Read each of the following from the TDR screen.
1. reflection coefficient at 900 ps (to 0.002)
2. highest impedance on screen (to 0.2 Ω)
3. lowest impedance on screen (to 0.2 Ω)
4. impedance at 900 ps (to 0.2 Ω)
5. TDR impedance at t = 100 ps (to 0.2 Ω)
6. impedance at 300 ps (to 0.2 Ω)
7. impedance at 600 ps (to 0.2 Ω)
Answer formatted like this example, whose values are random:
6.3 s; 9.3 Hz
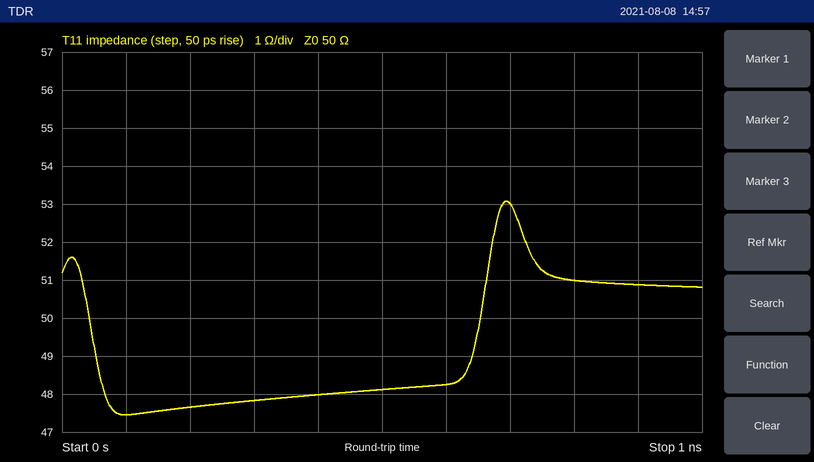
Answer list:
+0.008; 53.0 Ω; 47.4 Ω; 50.8 Ω; 47.4 Ω; 47.8 Ω; 48.2 Ω
